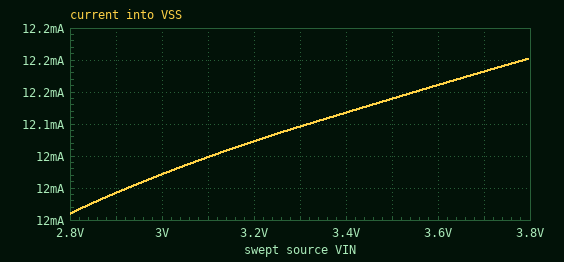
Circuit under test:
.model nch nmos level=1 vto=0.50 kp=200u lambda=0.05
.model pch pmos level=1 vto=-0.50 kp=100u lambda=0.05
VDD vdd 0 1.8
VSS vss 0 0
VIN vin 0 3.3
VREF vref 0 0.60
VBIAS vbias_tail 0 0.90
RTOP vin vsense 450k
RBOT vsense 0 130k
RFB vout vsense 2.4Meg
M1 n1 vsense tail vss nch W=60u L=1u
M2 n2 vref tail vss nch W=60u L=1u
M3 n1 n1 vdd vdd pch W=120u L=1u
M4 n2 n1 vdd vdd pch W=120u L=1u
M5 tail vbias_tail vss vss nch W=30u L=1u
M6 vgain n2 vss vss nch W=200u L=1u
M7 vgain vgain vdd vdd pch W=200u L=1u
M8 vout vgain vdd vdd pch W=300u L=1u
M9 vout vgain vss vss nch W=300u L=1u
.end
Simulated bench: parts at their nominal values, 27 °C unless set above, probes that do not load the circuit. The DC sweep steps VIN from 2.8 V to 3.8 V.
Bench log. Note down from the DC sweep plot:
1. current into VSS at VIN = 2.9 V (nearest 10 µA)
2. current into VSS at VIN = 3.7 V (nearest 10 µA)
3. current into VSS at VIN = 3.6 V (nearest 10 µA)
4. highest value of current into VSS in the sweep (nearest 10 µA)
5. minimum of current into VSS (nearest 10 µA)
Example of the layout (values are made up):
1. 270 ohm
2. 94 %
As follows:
1. 11.99 mA
2. 12.18 mA
3. 12.16 mA
4. 12.20 mA
5. 11.96 mA
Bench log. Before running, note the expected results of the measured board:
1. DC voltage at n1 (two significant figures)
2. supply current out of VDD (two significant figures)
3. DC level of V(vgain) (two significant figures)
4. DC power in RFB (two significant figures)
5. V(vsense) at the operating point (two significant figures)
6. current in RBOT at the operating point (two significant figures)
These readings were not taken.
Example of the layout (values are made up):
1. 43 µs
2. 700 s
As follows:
1. 1.1 V
2. 12 mA
3. 250 mV
4. 430 nW
5. 780 mV
6. 6.0 µA
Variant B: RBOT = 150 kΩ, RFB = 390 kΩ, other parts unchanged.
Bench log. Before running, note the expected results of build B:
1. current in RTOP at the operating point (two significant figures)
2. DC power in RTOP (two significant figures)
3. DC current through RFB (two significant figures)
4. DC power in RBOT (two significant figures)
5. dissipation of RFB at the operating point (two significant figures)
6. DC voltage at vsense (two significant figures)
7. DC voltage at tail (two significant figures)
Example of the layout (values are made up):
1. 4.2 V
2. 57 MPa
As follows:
1. 5.0 µA
2. 11 µW
3. 1.9 µA
4. 7.3 µW
5. 1.5 µW
6. 1.0 V
7. 280 mV
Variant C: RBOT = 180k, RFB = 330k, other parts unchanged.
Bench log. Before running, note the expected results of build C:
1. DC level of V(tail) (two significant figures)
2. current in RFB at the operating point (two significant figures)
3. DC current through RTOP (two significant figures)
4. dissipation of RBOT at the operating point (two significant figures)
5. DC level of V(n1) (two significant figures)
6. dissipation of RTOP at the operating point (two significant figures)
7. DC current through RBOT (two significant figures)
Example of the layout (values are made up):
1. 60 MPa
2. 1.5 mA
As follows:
1. 400 mV
2. 1.9 µA
3. 4.7 µA
4. 7.8 µW
5. 1.0 V
6. 10 µW
7. 6.6 µA
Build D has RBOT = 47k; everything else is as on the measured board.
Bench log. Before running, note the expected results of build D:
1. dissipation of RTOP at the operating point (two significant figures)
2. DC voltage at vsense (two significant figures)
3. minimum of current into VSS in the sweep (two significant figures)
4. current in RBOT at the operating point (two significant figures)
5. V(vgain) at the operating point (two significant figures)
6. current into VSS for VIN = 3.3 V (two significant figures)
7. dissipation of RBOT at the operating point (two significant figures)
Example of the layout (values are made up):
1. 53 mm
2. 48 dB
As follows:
1. 20 µW
2. 310 mV
3. 110 nA
4. 6.5 µA
5. 1.3 V
6. 130 nA
7. 2.0 µW
